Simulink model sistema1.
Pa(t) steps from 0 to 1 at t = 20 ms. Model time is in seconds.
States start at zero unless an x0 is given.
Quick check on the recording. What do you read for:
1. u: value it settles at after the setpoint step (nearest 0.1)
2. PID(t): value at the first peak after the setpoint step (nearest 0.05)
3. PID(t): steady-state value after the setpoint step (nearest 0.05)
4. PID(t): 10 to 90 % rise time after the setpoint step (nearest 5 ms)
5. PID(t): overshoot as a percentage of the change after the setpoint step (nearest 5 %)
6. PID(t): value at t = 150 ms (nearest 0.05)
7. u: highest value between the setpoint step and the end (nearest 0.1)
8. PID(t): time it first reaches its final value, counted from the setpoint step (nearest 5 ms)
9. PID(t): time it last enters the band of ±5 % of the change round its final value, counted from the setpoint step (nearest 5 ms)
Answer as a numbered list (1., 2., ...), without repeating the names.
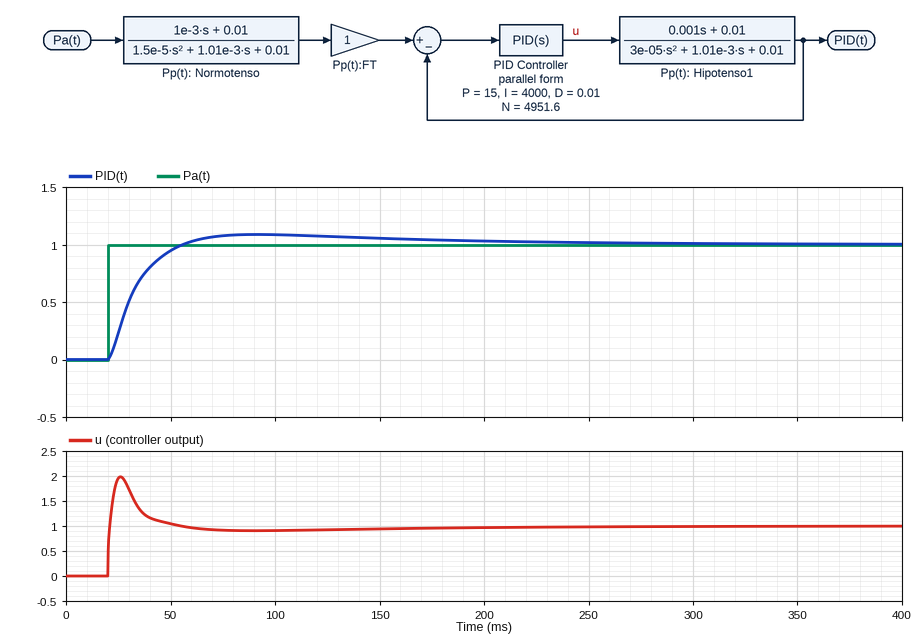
1. 1.0
2. 1.10
3. 1.00
4. 25 ms
5. 10 %
6. 1.05
7. 2.0
8. 35 ms
9. 135 ms
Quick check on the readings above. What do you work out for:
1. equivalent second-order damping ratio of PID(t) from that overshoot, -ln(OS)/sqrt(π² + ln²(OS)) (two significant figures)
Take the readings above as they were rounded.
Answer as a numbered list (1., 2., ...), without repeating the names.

1. 0.59
